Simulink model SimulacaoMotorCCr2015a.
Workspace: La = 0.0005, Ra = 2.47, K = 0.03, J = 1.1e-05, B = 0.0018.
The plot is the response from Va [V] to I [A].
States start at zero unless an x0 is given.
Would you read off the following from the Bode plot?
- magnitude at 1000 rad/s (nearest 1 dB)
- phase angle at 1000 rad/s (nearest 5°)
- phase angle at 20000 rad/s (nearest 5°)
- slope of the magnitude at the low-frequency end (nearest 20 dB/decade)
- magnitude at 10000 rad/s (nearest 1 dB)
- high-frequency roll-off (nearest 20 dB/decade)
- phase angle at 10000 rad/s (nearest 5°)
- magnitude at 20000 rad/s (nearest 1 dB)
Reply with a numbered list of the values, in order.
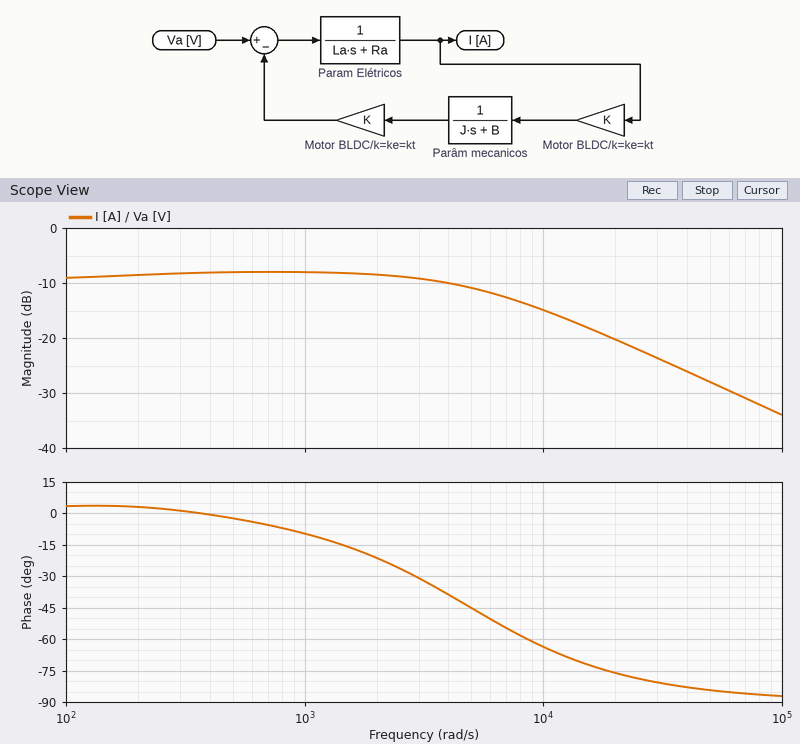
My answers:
1. -8 dB
2. -10°
3. -75°
4. 0 dB/decade
5. -15 dB
6. -20 dB/decade
7. -65°
8. -20 dB
